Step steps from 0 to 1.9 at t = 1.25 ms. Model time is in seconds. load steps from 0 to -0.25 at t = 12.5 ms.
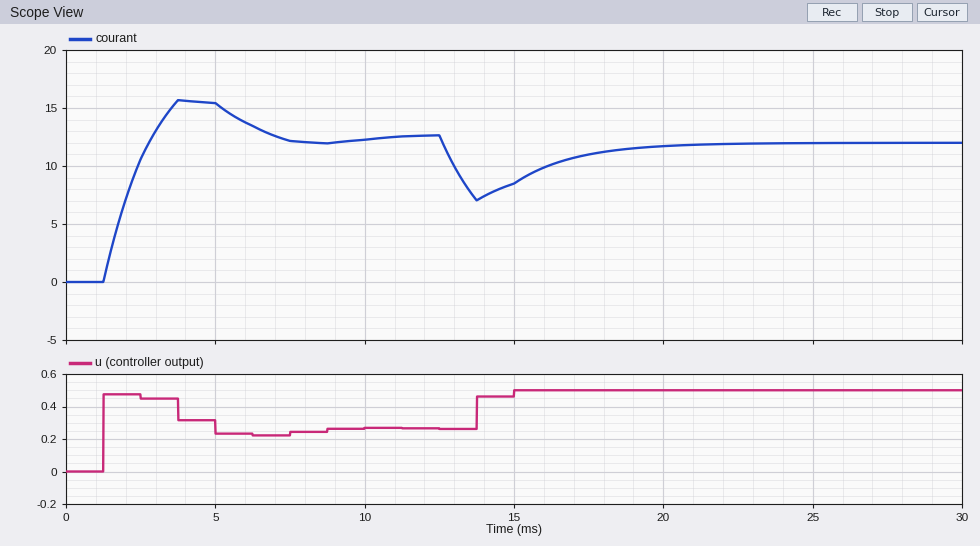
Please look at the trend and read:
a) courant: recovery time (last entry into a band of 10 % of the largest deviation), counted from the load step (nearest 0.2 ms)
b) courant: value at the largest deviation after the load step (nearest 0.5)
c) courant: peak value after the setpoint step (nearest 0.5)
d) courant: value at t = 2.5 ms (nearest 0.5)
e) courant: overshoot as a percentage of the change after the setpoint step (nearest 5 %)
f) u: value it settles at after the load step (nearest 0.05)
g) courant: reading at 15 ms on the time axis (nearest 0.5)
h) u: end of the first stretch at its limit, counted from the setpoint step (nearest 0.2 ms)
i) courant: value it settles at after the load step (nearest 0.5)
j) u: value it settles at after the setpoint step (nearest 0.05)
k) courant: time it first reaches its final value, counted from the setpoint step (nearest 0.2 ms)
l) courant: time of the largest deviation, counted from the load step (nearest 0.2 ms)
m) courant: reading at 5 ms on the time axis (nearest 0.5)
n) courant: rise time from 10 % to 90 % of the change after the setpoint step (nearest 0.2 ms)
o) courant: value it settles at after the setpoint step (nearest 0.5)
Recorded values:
6.2 ms
7.0
15.5
10.5
25 %
0.50
8.5
1.2 ms
12.0
0.25
1.6 ms
1.2 ms
15.5
1.2 ms
12.5
